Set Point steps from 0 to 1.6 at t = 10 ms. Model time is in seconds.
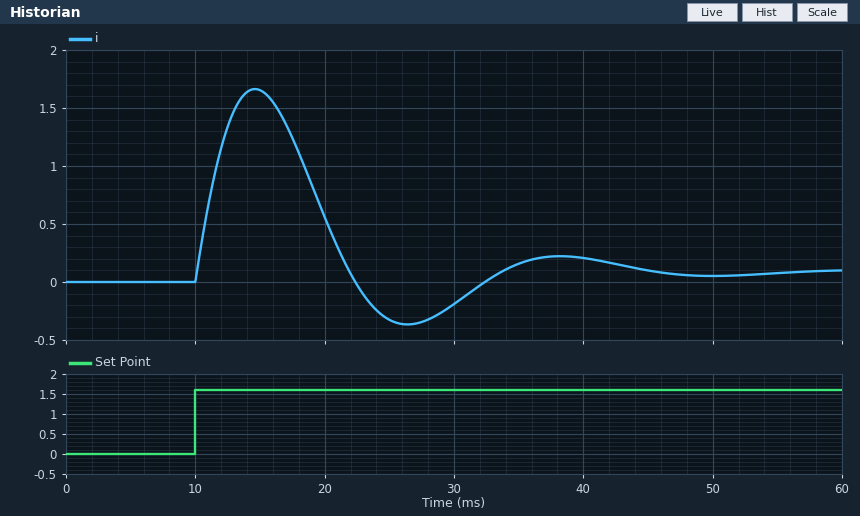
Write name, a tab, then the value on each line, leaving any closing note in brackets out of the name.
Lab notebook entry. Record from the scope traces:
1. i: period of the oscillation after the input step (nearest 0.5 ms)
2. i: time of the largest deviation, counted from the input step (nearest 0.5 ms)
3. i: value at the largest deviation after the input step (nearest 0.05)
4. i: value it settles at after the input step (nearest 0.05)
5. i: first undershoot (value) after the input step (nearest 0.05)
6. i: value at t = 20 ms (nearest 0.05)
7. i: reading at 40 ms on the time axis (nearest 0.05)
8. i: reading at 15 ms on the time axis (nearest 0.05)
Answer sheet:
i: period of the oscillation after the input step	23.5 ms
i: time of the largest deviation, counted from the input step	4.5 ms
i: value at the largest deviation after the input step	1.65
i: value it settles at after the input step	0.10
i: first undershoot (value) after the input step	-0.35
i: value at t = 20 ms	0.55
i: reading at 40 ms on the time axis	0.20
i: reading at 15 ms on the time axis	1.65
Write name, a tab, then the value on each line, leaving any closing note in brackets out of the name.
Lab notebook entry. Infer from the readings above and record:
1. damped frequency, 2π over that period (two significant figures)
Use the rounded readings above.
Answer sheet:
damped frequency, 2π over that period	0.27 rad/ms
